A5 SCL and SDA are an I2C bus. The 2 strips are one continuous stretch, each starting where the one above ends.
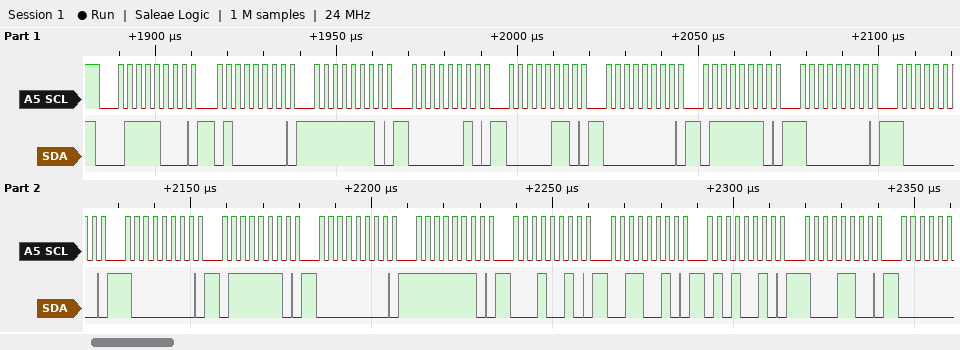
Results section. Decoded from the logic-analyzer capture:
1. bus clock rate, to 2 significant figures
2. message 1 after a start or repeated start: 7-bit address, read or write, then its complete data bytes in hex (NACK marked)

400 kHz
0x3C write: 40 FE 02 06 00 7E 80 80 80 7E 00 FE 12 32 52 8C
